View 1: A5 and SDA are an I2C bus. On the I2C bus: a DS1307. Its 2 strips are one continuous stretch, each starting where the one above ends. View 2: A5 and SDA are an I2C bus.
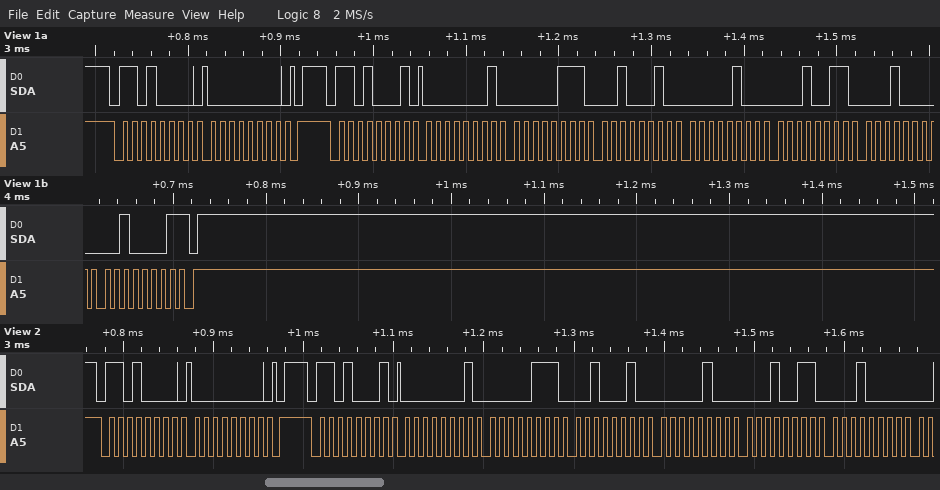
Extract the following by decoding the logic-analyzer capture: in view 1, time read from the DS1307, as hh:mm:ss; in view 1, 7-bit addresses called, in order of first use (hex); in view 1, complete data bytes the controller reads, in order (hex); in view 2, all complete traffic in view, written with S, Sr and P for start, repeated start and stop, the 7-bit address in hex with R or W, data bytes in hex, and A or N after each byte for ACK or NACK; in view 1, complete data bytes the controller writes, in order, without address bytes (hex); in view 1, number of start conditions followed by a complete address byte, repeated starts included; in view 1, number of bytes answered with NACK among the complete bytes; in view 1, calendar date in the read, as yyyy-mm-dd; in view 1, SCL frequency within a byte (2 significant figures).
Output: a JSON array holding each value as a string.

["22:07:01", "0x68", "01 07 22 04 13 10 21", "S 68W A 00 A P S 68R A 01 A 07 A 22 A 04 A 13 A 10 A", "00", "2", "1", "2021-10-13", "100 kHz"]
